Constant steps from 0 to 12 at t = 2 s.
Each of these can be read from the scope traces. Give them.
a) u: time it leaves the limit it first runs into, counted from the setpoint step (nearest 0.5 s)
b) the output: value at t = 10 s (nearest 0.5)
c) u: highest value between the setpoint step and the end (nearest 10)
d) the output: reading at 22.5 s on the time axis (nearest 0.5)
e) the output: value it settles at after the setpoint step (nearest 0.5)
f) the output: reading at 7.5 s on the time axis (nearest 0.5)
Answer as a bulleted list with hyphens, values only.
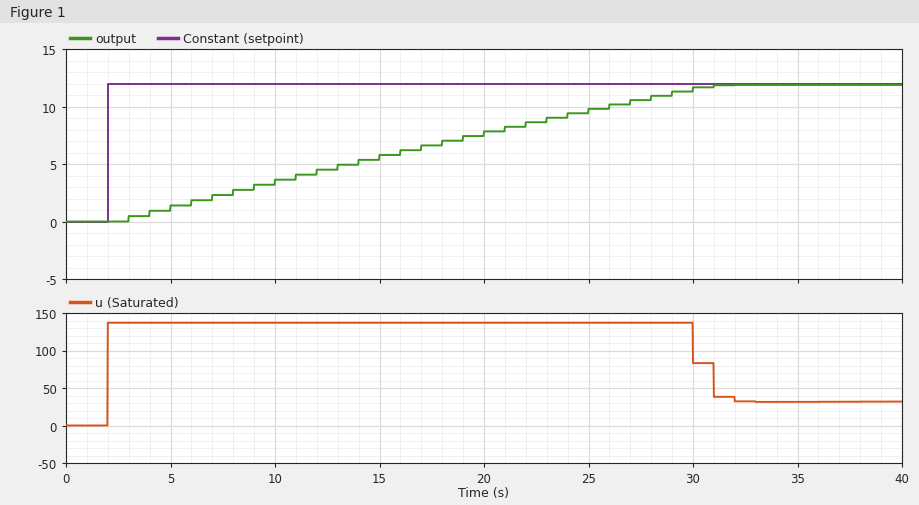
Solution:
- 28.0 s
- 3.5
- 140
- 8.5
- 12.0
- 2.5
